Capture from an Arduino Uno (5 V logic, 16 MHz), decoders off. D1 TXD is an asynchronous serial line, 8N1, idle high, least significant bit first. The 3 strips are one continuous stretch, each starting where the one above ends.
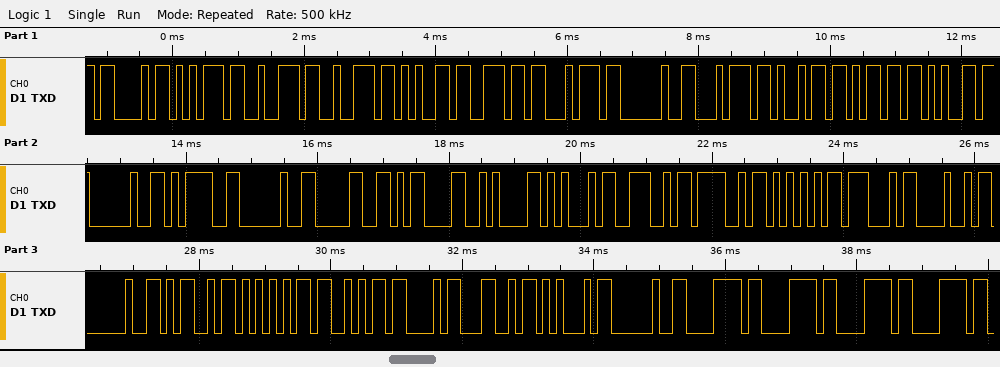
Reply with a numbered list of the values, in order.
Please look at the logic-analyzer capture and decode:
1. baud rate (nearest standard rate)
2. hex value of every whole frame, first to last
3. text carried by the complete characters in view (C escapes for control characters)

1. 9600 baud
2. 43 75 72 72 65 6E 74 20 74 69 6D 65 20 3D 20 30 0D 0A 45 4E 4F 55 47 48 20 4D 55 53 43 4C 45 20 78 78 78 78
3. "Current time = 0\r\nENOUGH MUSCLE xxxx"
